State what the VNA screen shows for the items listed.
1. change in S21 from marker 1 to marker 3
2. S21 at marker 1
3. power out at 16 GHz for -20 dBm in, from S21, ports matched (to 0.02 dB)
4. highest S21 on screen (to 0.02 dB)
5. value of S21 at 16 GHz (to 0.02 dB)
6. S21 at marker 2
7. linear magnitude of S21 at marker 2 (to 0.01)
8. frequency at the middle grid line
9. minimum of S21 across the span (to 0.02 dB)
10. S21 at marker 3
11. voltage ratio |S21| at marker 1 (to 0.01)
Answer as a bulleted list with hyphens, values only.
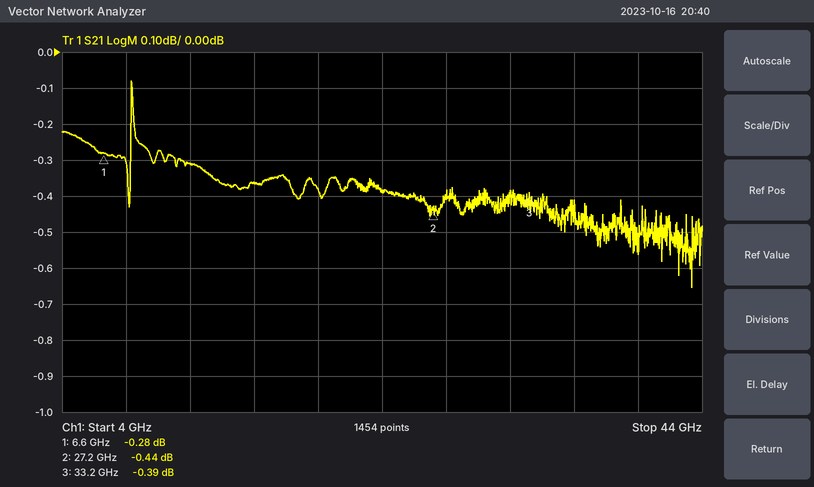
- -0.11 dB
- -0.28 dB
- -20.36 dBm
- -0.08 dB
- -0.36 dB
- -0.44 dB
- 0.95
- 24 GHz
- -0.66 dB
- -0.39 dB
- 0.97
